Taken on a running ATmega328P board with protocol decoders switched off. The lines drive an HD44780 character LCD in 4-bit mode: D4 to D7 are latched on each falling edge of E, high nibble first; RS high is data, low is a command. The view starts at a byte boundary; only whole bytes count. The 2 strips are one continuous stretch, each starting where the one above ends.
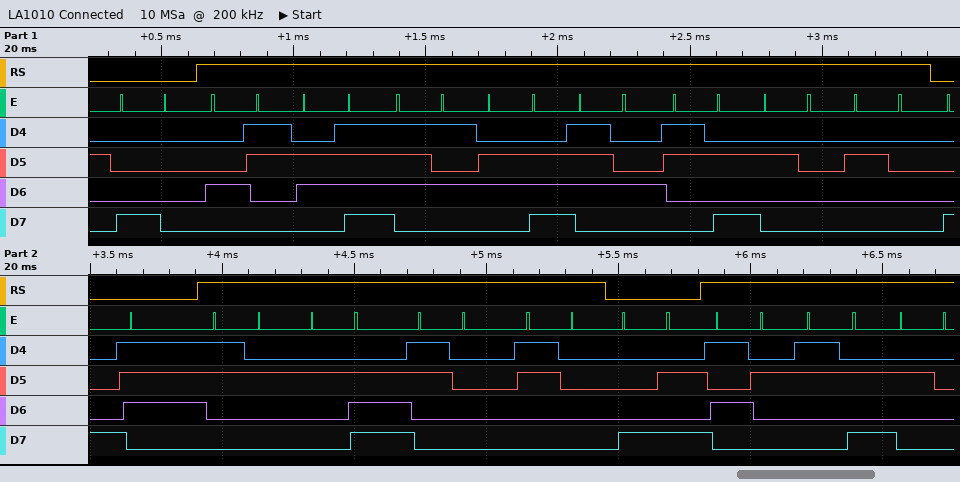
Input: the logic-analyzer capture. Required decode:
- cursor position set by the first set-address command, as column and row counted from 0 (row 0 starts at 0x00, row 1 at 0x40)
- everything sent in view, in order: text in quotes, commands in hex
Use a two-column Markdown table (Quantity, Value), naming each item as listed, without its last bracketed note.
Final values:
| Quantity | Value |
|---|---|
| cursor position set by the first set-address command, as column and row counted from 0 | column 0, row 0 |
| everything sent in view, in order: text in quotes, commands in hex | 0x80 "Count:  " 0x87 "2.00" 0x8A "R: " |
